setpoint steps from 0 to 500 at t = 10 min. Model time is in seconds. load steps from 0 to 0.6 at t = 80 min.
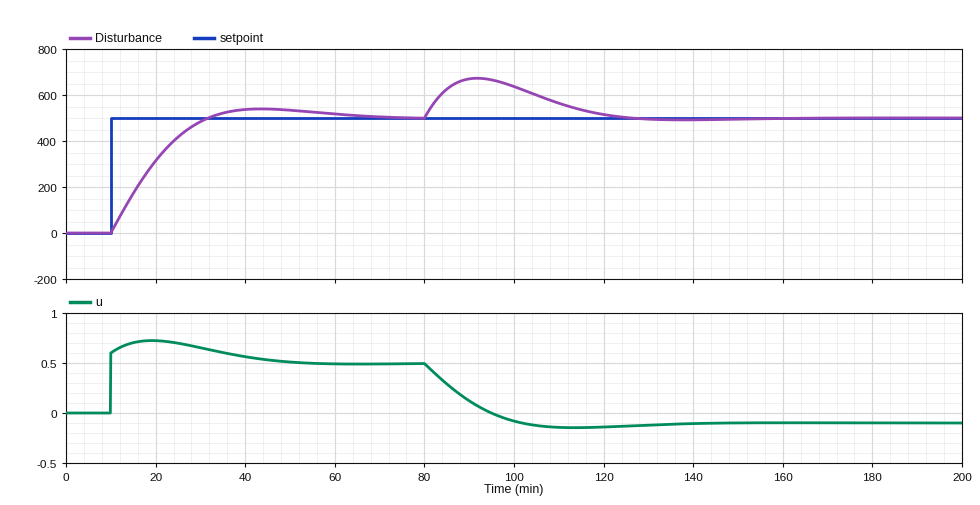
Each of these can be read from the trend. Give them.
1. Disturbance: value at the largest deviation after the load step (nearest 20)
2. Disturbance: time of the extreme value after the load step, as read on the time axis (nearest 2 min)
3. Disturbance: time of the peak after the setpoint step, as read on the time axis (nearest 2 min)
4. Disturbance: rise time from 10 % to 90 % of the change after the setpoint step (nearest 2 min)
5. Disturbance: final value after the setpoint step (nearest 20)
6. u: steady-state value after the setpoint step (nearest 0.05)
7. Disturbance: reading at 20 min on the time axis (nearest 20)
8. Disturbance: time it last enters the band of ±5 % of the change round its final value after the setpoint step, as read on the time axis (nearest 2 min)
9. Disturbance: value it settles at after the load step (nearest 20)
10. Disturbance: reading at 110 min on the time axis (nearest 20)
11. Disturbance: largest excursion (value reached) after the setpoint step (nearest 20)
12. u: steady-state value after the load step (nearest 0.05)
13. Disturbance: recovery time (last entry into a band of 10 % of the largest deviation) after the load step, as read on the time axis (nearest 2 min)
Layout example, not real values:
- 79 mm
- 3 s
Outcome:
- 680
- 92 min
- 44 min
- 16 min
- 500
- 0.50
- 320
- 56 min
- 500
- 560
- 540
- -0.10
- 120 min
